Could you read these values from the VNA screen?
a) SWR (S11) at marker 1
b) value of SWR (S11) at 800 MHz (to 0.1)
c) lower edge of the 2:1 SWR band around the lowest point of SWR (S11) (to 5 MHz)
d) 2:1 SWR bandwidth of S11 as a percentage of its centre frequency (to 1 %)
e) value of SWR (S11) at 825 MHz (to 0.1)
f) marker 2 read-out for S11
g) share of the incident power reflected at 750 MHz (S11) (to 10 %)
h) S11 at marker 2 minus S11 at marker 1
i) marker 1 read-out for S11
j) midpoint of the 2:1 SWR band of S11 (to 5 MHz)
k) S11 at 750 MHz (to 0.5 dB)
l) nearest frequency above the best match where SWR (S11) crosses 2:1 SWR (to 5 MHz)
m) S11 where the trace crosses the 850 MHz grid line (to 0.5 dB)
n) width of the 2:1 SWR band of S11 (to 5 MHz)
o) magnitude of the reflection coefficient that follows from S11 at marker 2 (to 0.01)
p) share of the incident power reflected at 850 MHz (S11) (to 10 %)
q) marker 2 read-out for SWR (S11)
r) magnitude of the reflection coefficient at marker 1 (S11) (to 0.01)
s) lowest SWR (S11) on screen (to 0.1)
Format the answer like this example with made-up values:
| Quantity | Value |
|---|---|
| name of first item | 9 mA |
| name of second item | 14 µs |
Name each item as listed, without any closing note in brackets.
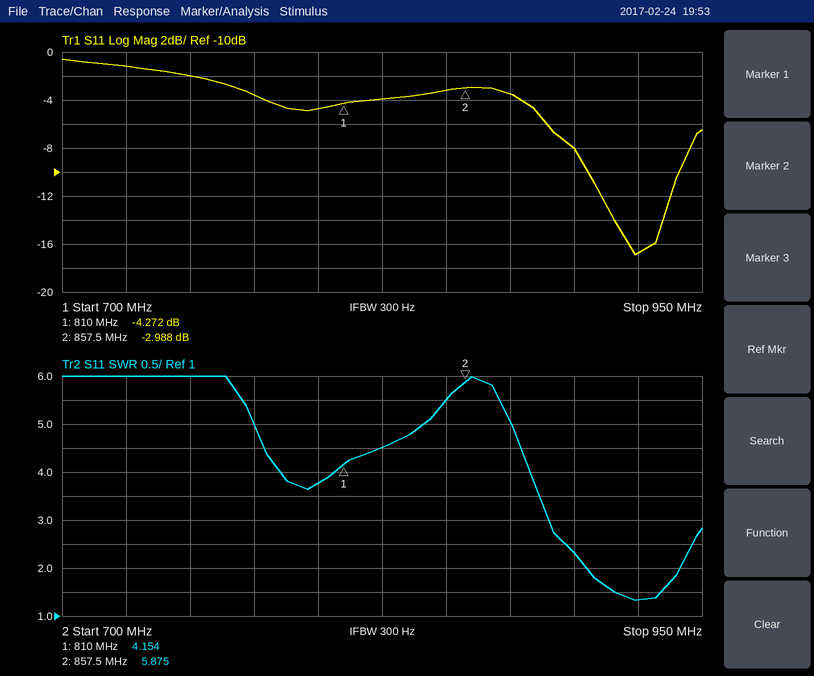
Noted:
| Quantity | Value |
|---|---|
| SWR (S11) at marker 1 | 4.154 |
| value of SWR (S11) at 800 MHz | 3.8 |
| lower edge of the 2:1 SWR band around the lowest point of SWR (S11) | 905 MHz |
| 2:1 SWR bandwidth of S11 as a percentage of its centre frequency | 4 % |
| value of SWR (S11) at 825 MHz | 4.5 |
| marker 2 read-out for S11 | -2.988 dB |
| share of the incident power reflected at 750 MHz (S11) | 60 % |
| S11 at marker 2 minus S11 at marker 1 | 1.284 dB |
| marker 1 read-out for S11 | -4.272 dB |
| midpoint of the 2:1 SWR band of S11 | 925 MHz |
| S11 at 750 MHz | -2.0 dB |
| nearest frequency above the best match where SWR (S11) crosses 2:1 SWR | 940 MHz |
| S11 where the trace crosses the 850 MHz grid line | -3.0 dB |
| width of the 2:1 SWR band of S11 | 35 MHz |
| magnitude of the reflection coefficient that follows from S11 at marker 2 | 0.71 |
| share of the incident power reflected at 850 MHz (S11) | 50 % |
| marker 2 read-out for SWR | 5.875 |
| magnitude of the reflection coefficient at marker 1 (S11) | 0.61 |
| lowest SWR (S11) on screen | 1.3 |
